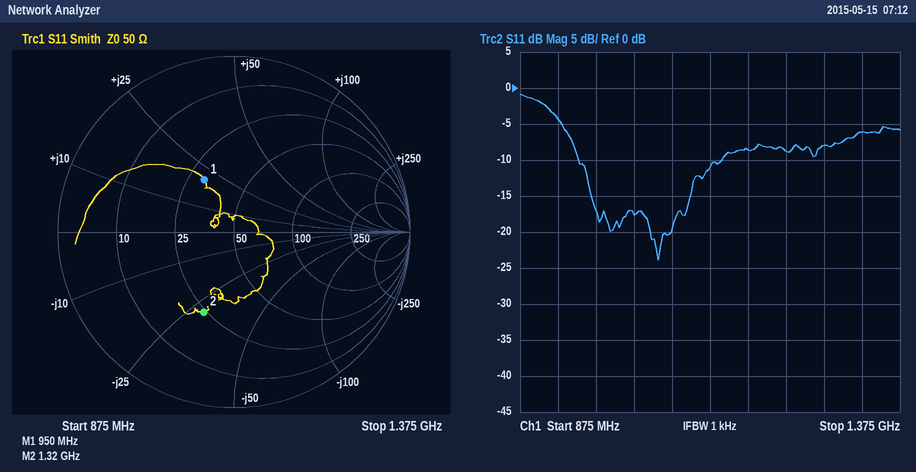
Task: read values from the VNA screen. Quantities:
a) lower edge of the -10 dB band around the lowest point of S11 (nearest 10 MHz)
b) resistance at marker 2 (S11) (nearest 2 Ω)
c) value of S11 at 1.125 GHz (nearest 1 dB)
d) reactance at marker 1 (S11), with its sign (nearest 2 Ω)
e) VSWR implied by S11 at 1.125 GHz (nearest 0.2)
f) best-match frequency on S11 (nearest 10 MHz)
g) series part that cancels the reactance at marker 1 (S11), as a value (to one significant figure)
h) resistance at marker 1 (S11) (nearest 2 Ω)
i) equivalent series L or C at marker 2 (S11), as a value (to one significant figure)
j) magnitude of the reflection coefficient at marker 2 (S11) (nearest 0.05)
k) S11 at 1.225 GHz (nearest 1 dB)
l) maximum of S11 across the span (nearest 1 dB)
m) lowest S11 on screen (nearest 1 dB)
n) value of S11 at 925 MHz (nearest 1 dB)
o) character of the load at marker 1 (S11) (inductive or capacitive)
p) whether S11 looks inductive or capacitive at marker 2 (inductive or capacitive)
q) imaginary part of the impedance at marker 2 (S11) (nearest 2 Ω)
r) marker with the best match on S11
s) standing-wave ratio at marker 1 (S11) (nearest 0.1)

950 MHz
24 Ω
-11 dB
+20 Ω
1.8
1.06 GHz
8 pF
30 Ω
4 pF
0.50
-9 dB
-1 dB
-24 dB
-4 dB
inductive
capacitive
-28 Ω
marker 1
2.0
